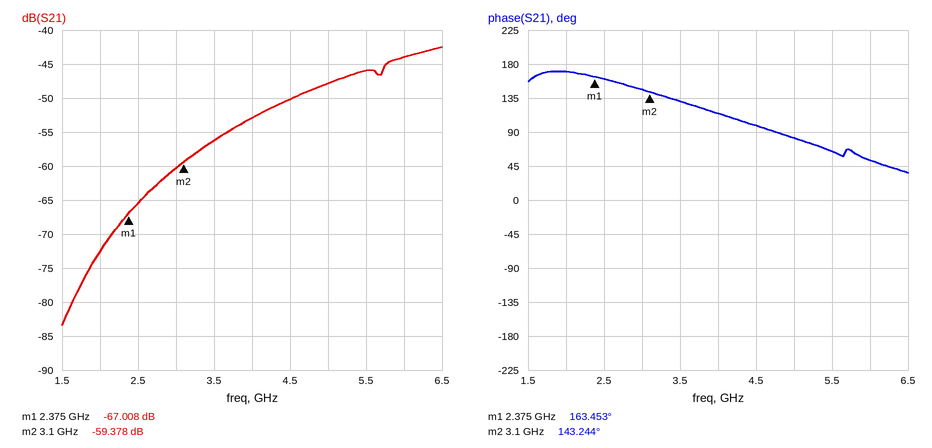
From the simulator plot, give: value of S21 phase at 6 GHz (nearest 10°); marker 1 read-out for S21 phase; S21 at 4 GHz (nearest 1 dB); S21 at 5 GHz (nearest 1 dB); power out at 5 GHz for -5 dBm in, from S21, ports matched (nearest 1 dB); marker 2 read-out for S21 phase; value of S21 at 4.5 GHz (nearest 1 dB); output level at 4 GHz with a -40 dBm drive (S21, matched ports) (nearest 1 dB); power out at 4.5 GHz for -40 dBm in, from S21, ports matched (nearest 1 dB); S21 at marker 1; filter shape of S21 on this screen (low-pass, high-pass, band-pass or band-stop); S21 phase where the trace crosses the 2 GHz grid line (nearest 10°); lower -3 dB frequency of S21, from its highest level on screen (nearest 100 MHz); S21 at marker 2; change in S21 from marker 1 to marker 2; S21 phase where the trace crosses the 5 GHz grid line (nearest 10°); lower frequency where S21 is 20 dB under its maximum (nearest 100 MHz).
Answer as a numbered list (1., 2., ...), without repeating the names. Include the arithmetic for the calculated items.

1. 50°
2. 163.453°
3. -53 dB
4. -48 dB
5. -5 dBm + (-48 dB) = -53 dBm
6. 143.244°
7. -50 dB
8. -40 dBm + (-53 dB) = -93 dBm
9. -40 dBm + (-50 dB) = -90 dBm
10. -67.008 dB
11. high-pass
12. 170°
13. 5.7 GHz
14. -59.378 dB
15. -59.378 − (-67.008) = 7.630 dB
16. 80°
17. 2.8 GHz
